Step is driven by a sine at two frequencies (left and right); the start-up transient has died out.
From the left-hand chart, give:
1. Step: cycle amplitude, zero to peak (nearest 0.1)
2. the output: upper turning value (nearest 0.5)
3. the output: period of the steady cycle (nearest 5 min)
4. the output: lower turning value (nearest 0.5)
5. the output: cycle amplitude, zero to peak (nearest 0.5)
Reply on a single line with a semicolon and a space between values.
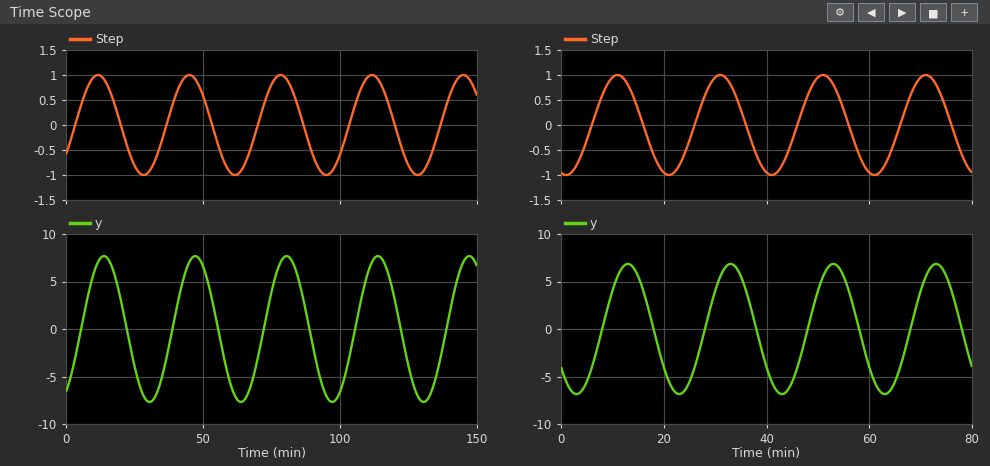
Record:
1.0; 7.5; 35 min; -7.5; 7.5
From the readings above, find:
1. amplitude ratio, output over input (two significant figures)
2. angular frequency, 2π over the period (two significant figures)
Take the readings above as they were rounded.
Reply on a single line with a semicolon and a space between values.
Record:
7.5; 0.18 rad/min
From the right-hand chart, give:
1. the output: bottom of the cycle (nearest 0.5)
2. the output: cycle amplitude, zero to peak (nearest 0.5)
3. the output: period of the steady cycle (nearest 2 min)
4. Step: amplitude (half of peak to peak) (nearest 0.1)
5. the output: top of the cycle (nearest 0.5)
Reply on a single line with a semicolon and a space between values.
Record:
-7.0; 7.0; 20 min; 1.0; 7.0
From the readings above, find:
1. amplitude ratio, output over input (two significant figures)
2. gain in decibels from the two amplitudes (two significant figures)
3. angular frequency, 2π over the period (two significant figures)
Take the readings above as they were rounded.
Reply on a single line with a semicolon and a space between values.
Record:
7.0; 17 dB; 0.31 rad/min
